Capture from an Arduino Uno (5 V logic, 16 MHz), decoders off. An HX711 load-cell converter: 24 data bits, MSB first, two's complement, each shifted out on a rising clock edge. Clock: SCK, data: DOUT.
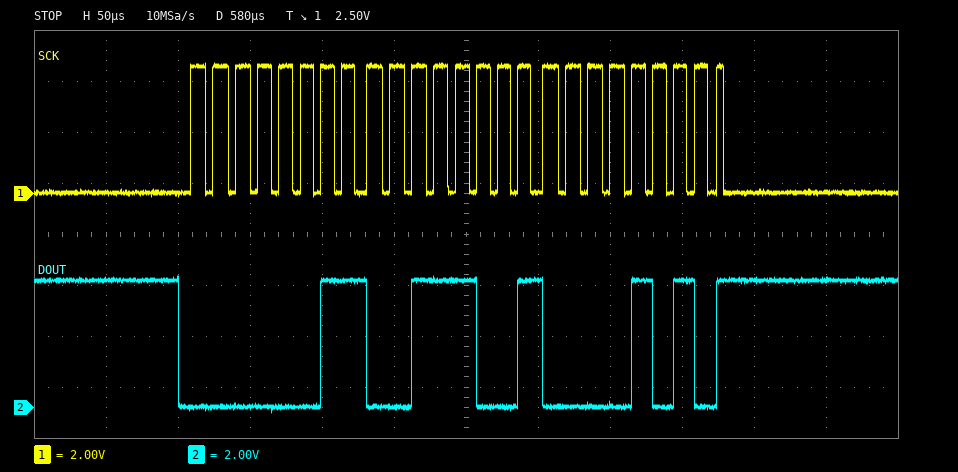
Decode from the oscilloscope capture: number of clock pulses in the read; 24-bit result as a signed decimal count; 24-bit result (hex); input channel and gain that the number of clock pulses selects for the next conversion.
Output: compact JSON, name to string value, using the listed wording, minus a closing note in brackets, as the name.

{"number of clock pulses in the read": "25", "24-bit result as a signed decimal count": "211210", "24-bit result": "0x03390A", "input channel and gain that the number of clock pulses selects for the next conversion": "channel A, gain 128"}
